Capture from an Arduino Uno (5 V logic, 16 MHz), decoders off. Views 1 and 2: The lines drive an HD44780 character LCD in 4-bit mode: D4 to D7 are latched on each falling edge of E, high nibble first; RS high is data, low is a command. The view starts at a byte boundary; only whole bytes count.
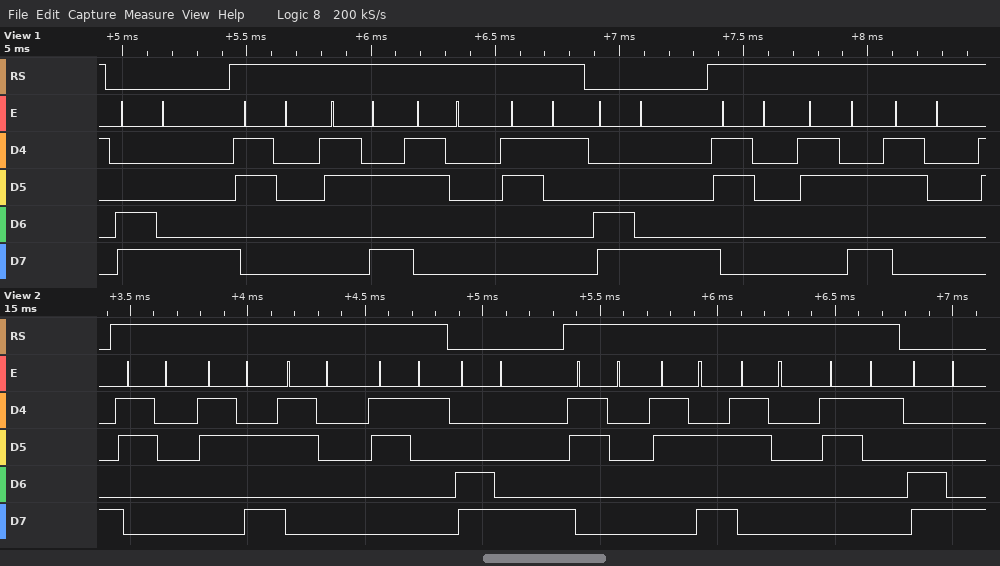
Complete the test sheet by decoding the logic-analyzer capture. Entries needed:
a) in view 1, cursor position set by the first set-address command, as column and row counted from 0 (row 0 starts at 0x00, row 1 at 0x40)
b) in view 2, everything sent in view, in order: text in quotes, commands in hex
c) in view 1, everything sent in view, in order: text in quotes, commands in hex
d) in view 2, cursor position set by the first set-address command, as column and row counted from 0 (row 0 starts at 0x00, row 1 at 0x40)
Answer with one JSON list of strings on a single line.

["column 8, row 1", "\"0:01\" 0xC8 \"0:01\" 0xC8", "0xC8 \"0:01\" 0xC8 \"0:0\"", "column 8, row 1"]
